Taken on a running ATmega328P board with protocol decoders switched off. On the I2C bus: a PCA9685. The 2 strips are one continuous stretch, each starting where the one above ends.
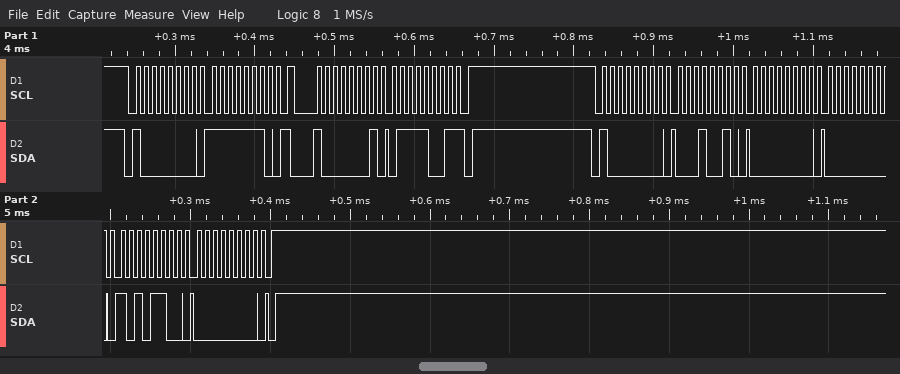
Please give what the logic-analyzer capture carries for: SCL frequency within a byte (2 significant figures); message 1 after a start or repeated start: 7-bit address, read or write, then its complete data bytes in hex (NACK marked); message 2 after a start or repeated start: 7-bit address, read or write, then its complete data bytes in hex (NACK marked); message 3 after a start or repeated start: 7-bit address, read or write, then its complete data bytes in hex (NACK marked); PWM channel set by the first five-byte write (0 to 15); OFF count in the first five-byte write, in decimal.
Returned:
100 kHz
0x40 write: FE
0x40 read: 79 NACK
0x40 write: 12 00 00 AC 00
3
172
